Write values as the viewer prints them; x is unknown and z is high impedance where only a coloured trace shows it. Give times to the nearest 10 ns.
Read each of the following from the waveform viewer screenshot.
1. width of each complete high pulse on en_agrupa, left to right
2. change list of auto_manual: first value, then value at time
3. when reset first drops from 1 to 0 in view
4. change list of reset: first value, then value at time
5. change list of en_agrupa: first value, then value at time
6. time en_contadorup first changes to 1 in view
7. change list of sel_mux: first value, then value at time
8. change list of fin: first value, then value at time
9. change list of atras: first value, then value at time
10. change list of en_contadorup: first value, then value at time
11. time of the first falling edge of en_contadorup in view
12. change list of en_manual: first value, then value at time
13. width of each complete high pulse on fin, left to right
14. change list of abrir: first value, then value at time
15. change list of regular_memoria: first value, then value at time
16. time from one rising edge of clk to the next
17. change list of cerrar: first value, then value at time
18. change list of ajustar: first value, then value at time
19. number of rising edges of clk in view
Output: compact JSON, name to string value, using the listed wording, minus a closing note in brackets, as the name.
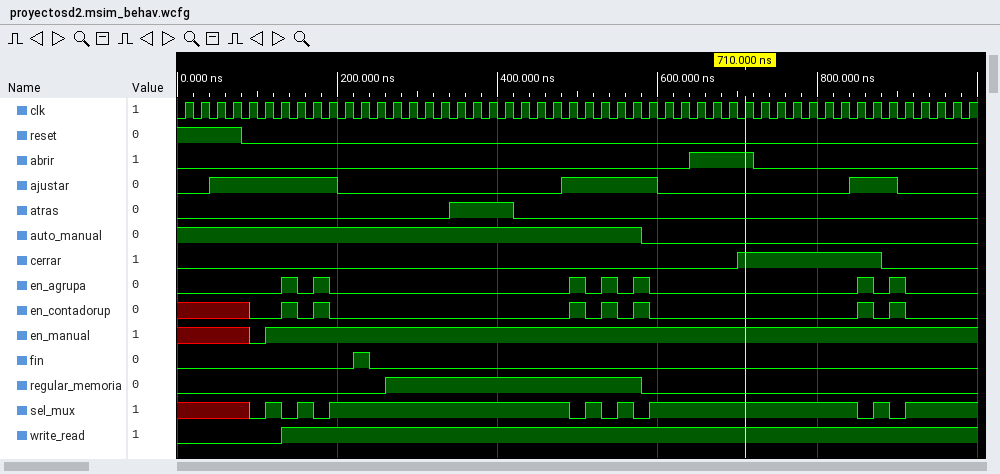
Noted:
{"width of each complete high pulse on en_agrupa, left to right": "20 ns, 20 ns, 20 ns, 20 ns, 20 ns, 20 ns, 20 ns", "change list of auto_manual: first value, then value at time": "1, 0 at 580 ns", "when reset first drops from 1 to 0 in view": "80 ns", "change list of reset: first value, then value at time": "1, 0 at 80 ns", "change list of en_agrupa: first value, then value at time": "0, 1 at 130 ns, 0 at 150 ns, 1 at 170 ns, 0 at 190 ns, 1 at 490 ns, 0 at 510 ns, 1 at 530 ns, 0 at 550 ns, 1 at 570 ns, 0 at 590 ns, 1 at 850 ns, 0 at 870 ns, 1 at 890 ns, 0 at 910 ns", "time en_contadorup first changes to 1 in view": "130 ns", "change list of sel_mux: first value, then value at time": "x, 0 at 90 ns, 1 at 110 ns, 0 at 130 ns, 1 at 150 ns, 0 at 170 ns, 1 at 190 ns, 0 at 490 ns, 1 at 510 ns, 0 at 530 ns, 1 at 550 ns, 0 at 570 ns, 1 at 590 ns, 0 at 850 ns, 1 at 870 ns, 0 at 890 ns, 1 at 910 ns", "change list of fin: first value, then value at time": "0, 1 at 220 ns, 0 at 240 ns", "change list of atras: first value, then value at time": "0, 1 at 340 ns, 0 at 420 ns", "change list of en_contadorup: first value, then value at time": "x, 0 at 90 ns, 1 at 130 ns, 0 at 150 ns, 1 at 170 ns, 0 at 190 ns, 1 at 490 ns, 0 at 510 ns, 1 at 530 ns, 0 at 550 ns, 1 at 570 ns, 0 at 590 ns, 1 at 850 ns, 0 at 870 ns, 1 at 890 ns, 0 at 910 ns", "time of the first falling edge of en_contadorup in view": "150 ns", "change list of en_manual: first value, then value at time": "x, 0 at 90 ns, 1 at 110 ns", "width of each complete high pulse on fin, left to right": "20 ns", "change list of abrir: first value, then value at time": "0, 1 at 640 ns, 0 at 720 ns", "change list of regular_memoria: first value, then value at time": "0, 1 at 260 ns, 0 at 580 ns", "time from one rising edge of clk to the next": "20 ns", "change list of cerrar: first value, then value at time": "0, 1 at 700 ns, 0 at 880 ns", "change list of ajustar: first value, then value at time": "0, 1 at 40 ns, 0 at 200 ns, 1 at 480 ns, 0 at 600 ns, 1 at 840 ns, 0 at 900 ns", "number of rising edges of clk in view": "50"}
